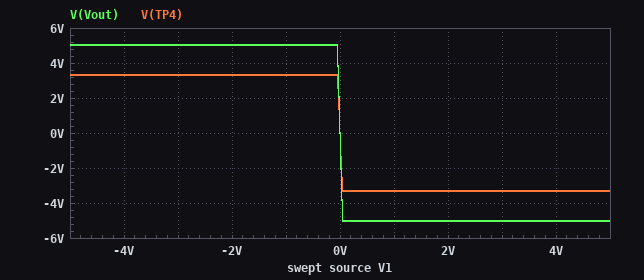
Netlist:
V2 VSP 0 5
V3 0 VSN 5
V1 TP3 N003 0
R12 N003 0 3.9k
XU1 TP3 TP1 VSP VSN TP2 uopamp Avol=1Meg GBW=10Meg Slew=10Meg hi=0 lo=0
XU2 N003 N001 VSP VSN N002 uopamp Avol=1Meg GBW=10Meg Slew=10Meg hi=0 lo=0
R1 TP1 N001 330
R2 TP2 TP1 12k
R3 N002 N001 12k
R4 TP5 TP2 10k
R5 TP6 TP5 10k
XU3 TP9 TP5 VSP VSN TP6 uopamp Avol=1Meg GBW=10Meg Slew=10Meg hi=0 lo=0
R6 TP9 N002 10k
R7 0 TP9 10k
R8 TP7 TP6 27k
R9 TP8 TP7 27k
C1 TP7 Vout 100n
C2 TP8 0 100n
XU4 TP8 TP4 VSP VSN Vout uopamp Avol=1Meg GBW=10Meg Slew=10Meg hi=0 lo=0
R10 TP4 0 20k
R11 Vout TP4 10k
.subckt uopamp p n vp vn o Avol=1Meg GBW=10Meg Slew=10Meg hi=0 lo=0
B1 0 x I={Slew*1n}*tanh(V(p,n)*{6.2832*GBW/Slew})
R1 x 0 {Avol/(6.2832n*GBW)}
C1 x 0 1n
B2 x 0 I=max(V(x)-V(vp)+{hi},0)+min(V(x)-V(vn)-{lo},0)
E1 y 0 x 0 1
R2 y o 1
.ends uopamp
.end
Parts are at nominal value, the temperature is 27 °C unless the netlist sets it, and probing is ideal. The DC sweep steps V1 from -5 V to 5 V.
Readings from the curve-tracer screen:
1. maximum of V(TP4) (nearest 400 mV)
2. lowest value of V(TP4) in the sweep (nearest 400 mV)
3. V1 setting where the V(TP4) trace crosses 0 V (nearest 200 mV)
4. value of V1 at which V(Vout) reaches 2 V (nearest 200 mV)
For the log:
3.2 V
-3.2 V
0 V
0 V
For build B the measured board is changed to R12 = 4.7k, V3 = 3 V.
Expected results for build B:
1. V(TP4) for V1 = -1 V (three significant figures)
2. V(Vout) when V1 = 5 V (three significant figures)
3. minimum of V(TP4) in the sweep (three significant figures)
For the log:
3.34 V
-3.01 V
-2.01 V
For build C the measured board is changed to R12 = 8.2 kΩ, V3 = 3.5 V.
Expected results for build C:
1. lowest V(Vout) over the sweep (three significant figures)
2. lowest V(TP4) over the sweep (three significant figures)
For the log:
-3.51 V
-2.34 V
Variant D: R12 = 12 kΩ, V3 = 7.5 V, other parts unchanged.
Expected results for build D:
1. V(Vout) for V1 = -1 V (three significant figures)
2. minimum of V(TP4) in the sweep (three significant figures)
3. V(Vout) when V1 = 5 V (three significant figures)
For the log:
5.01 V
-5.01 V
-7.51 V
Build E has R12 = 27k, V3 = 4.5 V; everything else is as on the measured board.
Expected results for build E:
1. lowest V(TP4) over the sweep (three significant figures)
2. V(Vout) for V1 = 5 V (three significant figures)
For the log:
-3.01 V
-4.51 V
